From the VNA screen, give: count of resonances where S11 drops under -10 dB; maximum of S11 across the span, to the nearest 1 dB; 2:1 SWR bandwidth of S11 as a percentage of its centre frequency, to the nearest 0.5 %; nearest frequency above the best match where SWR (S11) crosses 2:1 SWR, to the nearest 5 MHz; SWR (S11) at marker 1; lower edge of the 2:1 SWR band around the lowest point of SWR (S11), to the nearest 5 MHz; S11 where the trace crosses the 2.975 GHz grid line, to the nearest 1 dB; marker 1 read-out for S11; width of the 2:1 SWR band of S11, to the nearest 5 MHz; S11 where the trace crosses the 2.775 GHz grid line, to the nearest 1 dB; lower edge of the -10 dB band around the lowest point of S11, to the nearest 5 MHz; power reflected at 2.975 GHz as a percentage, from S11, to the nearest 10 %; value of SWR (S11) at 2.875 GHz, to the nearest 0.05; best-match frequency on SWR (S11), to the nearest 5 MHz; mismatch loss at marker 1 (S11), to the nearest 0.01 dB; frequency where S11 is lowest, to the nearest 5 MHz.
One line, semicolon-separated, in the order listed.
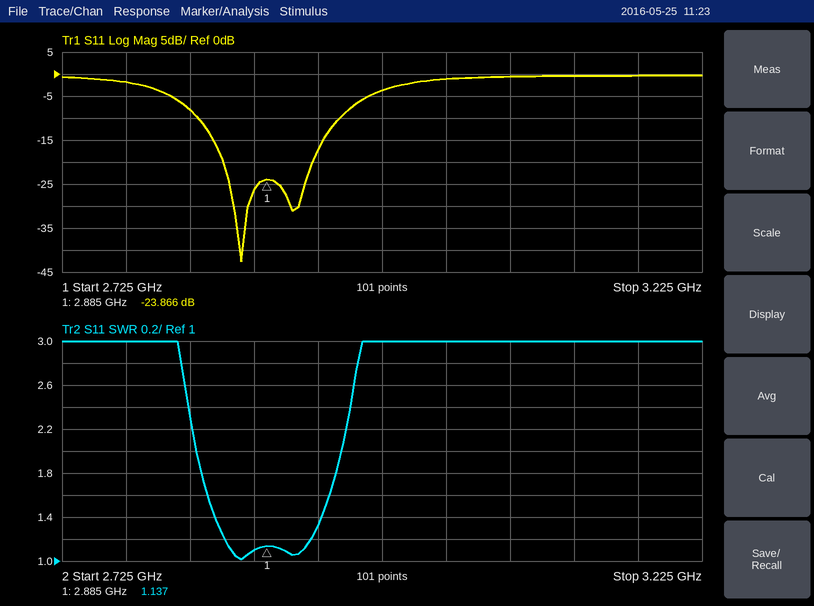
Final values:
2; 0 dB; 4.0 %; 2.945 GHz; 1.137; 2.830 GHz; -4 dB; -23.866 dB; 115 MHz; -2 dB; 2.830 GHz; 40 %; 1.10; 2.865 GHz; 0.02 dB; 2.865 GHz
